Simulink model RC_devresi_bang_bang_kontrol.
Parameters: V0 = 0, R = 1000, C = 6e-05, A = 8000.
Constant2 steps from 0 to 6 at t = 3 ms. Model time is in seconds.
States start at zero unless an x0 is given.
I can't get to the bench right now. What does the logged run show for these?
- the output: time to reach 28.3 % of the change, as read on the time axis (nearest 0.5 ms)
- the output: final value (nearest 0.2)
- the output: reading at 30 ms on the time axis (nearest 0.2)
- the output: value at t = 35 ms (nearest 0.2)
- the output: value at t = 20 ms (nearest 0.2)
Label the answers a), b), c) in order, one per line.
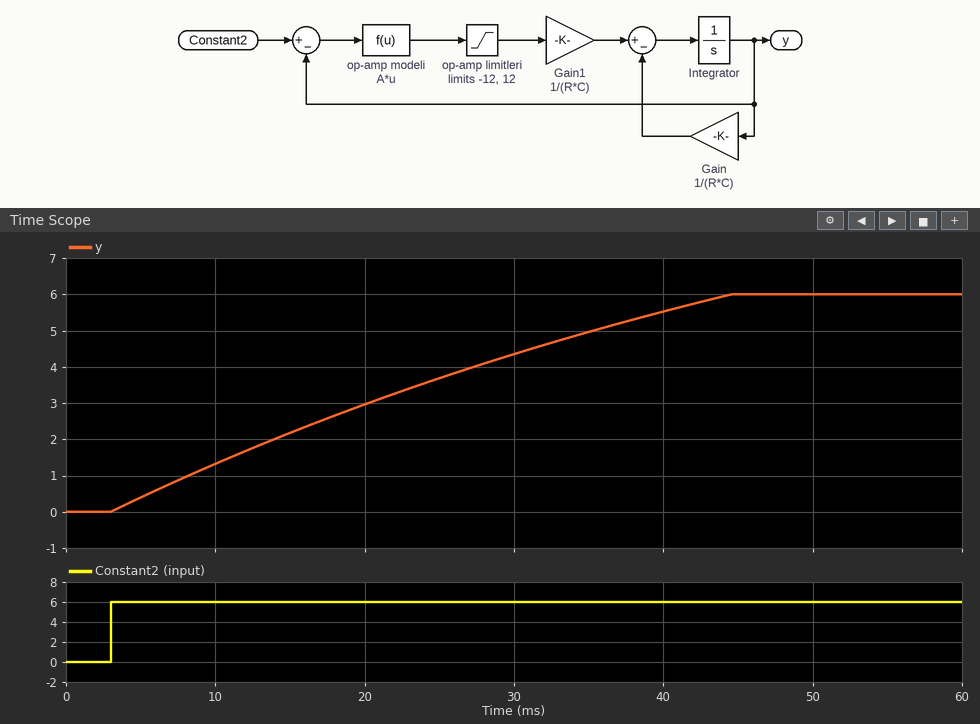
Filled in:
a) 12.0 ms
b) 6.0
c) 4.4
d) 5.0
e) 3.0
